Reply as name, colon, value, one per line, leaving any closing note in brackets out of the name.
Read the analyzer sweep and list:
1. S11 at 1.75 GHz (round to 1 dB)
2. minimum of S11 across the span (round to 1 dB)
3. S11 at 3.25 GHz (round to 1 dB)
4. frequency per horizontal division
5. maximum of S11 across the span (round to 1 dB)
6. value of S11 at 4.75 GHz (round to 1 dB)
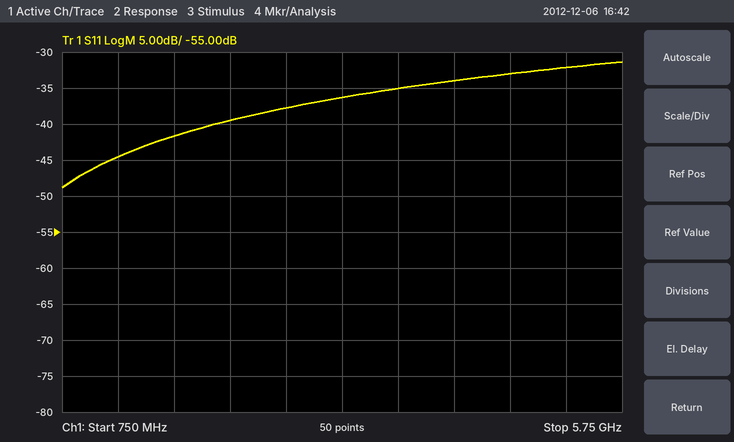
S11 at 1.75 GHz: -42 dB
minimum of S11 across the span: -49 dB
S11 at 3.25 GHz: -36 dB
frequency per horizontal division: 500 MHz
maximum of S11 across the span: -31 dB
value of S11 at 4.75 GHz: -33 dB
